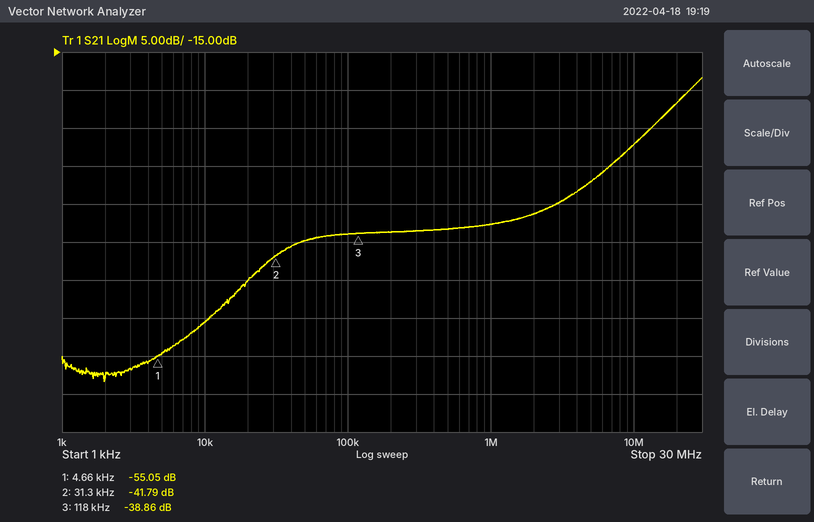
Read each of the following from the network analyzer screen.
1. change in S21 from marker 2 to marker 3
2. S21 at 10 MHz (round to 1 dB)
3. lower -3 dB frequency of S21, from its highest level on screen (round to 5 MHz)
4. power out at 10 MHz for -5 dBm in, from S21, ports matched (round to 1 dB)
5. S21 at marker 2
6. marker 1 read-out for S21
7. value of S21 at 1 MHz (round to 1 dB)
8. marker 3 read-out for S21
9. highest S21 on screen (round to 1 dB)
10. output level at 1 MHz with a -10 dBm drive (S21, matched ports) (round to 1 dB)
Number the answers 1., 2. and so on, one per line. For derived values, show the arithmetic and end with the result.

1. -38.86 − (-41.79) = 2.93 dB
2. -27 dB
3. 20 MHz
4. -5 dBm + (-27 dB) = -32 dBm
5. -41.79 dB
6. -55.05 dB
7. -38 dB
8. -38.86 dB
9. -18 dB
10. -10 dBm + (-38 dB) = -48 dBm
